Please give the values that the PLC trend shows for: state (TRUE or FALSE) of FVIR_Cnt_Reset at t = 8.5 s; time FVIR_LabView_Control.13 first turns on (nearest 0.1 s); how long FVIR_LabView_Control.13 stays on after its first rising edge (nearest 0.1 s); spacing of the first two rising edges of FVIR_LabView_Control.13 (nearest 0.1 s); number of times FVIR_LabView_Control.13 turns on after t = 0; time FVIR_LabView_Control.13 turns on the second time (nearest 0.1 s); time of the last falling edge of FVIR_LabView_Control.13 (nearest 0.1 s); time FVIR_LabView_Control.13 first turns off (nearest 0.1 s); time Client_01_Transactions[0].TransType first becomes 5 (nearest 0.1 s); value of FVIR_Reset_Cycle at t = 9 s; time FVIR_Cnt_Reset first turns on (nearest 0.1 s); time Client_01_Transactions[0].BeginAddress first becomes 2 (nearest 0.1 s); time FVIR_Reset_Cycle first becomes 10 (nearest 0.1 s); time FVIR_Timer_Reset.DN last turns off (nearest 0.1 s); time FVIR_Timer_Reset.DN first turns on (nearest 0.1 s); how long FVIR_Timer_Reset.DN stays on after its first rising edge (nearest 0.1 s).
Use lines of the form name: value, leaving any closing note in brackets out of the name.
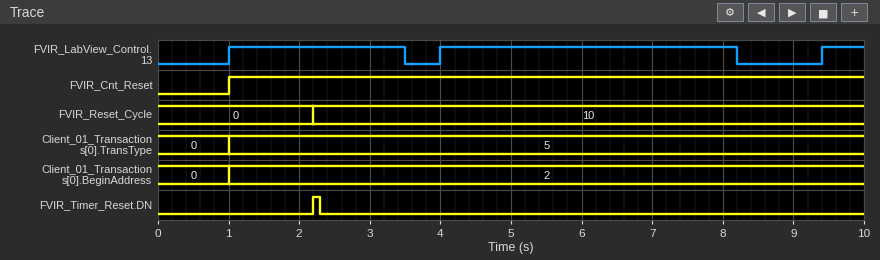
state (TRUE or FALSE) of FVIR_Cnt_Reset at t = 8.5 s: TRUE
time FVIR_LabView_Control.13 first turns on: 1.0 s
how long FVIR_LabView_Control.13 stays on after its first rising edge: 2.5 s
spacing of the first two rising edges of FVIR_LabView_Control.13: 3.0 s
number of times FVIR_LabView_Control.13 turns on after t = 0: 3
time FVIR_LabView_Control.13 turns on the second time: 4.0 s
time of the last falling edge of FVIR_LabView_Control.13: 8.2 s
time FVIR_LabView_Control.13 first turns off: 3.5 s
time Client_01_Transactions[0].TransType first becomes 5: 1.0 s
value of FVIR_Reset_Cycle at t = 9 s: 10
time FVIR_Cnt_Reset first turns on: 1.0 s
time Client_01_Transactions[0].BeginAddress first becomes 2: 1.0 s
time FVIR_Reset_Cycle first becomes 10: 2.2 s
time FVIR_Timer_Reset.DN last turns off: 2.3 s
time FVIR_Timer_Reset.DN first turns on: 2.2 s
how long FVIR_Timer_Reset.DN stays on after its first rising edge: 0.1 s
